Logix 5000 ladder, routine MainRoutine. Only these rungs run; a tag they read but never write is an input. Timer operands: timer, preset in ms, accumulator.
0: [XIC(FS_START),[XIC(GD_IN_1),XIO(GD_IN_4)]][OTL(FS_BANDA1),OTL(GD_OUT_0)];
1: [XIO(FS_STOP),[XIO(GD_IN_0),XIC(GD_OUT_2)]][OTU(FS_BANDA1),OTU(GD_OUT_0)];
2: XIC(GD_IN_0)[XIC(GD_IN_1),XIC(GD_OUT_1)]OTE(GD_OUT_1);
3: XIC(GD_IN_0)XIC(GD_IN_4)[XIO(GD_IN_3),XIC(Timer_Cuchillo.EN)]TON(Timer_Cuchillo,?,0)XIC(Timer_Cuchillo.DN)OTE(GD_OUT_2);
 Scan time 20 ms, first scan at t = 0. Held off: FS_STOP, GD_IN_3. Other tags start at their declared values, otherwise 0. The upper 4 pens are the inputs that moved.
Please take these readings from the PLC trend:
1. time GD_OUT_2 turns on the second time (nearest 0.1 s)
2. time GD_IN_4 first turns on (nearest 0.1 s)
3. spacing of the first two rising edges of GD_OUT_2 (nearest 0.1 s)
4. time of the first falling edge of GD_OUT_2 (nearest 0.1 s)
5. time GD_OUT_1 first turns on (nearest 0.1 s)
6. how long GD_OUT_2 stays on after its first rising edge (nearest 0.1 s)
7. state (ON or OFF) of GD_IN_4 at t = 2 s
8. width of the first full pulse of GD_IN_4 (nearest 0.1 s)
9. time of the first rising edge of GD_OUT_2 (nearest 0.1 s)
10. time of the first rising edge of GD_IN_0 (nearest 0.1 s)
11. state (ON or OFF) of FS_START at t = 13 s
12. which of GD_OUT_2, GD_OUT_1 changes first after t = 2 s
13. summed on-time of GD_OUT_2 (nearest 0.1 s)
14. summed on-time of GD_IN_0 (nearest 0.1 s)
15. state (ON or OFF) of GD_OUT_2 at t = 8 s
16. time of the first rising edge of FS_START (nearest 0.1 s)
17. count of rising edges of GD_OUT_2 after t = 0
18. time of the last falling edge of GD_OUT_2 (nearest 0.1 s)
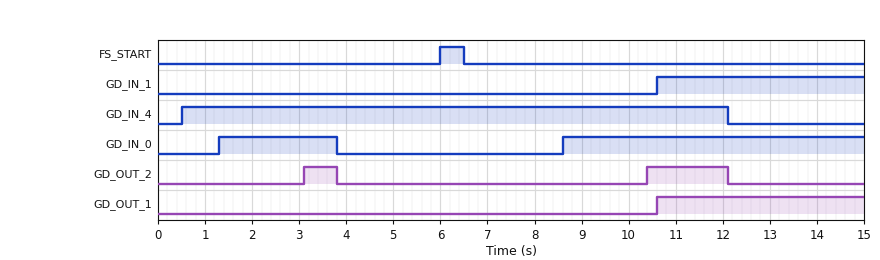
10.4 s
0.5 s
7.3 s
3.8 s
10.6 s
0.7 s
ON
11.6 s
3.1 s
1.3 s
OFF
GD_OUT_2
2.4 s
8.9 s
OFF
6.0 s
2
12.1 s
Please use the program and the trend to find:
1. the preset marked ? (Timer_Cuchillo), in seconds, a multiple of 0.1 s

1.8 s
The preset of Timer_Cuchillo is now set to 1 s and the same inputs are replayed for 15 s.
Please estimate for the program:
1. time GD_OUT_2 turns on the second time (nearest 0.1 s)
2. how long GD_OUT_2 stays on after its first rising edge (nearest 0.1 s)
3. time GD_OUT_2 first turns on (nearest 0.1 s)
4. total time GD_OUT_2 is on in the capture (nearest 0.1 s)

9.6 s
1.5 s
2.3 s
4.0 s
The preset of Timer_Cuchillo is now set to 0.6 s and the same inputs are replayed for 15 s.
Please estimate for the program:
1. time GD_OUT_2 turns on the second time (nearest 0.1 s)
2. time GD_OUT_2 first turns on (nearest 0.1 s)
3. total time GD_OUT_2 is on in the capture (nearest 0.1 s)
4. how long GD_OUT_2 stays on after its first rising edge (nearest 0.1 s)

9.2 s
1.9 s
4.8 s
1.9 s
